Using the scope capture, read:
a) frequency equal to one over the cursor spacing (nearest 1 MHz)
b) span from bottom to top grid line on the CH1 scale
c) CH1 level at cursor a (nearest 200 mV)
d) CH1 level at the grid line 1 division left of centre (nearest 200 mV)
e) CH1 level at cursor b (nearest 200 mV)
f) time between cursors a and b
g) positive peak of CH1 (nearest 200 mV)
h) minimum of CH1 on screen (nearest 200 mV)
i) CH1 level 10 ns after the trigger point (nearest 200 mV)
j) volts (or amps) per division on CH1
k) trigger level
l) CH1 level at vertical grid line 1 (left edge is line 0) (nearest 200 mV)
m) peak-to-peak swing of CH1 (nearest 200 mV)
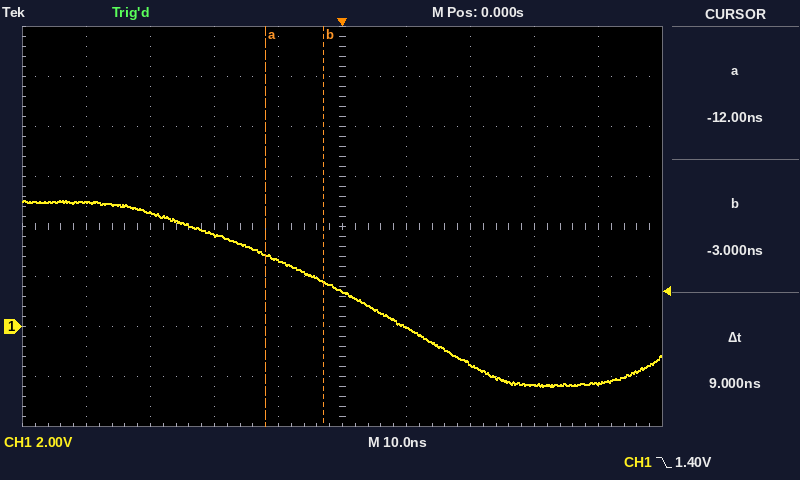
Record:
111 MHz
16 V
2.8 V
2.6 V
1.8 V
9 ns
5.0 V
-2.4 V
0.0 V
2 V
1.40 V
5.0 V
7.4 V
